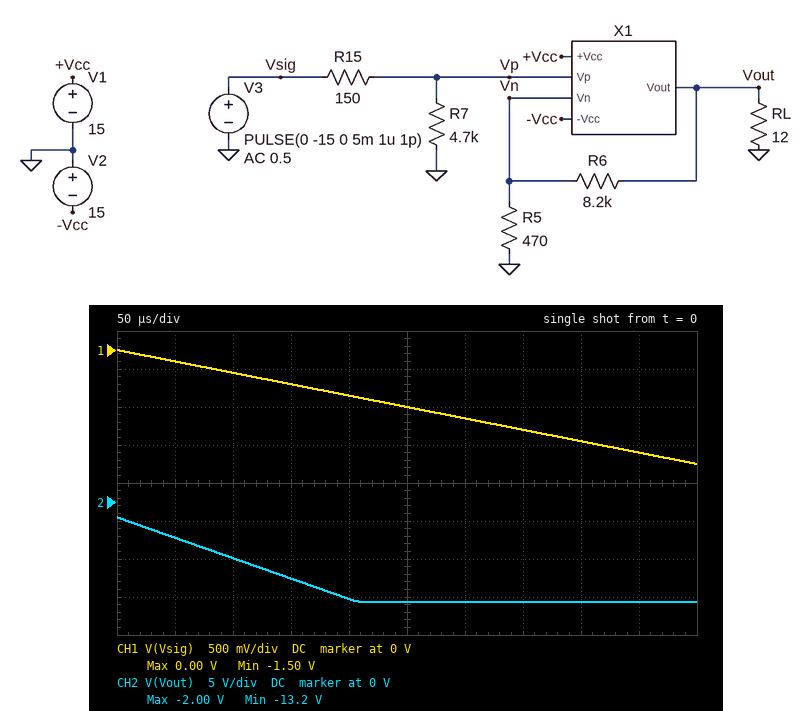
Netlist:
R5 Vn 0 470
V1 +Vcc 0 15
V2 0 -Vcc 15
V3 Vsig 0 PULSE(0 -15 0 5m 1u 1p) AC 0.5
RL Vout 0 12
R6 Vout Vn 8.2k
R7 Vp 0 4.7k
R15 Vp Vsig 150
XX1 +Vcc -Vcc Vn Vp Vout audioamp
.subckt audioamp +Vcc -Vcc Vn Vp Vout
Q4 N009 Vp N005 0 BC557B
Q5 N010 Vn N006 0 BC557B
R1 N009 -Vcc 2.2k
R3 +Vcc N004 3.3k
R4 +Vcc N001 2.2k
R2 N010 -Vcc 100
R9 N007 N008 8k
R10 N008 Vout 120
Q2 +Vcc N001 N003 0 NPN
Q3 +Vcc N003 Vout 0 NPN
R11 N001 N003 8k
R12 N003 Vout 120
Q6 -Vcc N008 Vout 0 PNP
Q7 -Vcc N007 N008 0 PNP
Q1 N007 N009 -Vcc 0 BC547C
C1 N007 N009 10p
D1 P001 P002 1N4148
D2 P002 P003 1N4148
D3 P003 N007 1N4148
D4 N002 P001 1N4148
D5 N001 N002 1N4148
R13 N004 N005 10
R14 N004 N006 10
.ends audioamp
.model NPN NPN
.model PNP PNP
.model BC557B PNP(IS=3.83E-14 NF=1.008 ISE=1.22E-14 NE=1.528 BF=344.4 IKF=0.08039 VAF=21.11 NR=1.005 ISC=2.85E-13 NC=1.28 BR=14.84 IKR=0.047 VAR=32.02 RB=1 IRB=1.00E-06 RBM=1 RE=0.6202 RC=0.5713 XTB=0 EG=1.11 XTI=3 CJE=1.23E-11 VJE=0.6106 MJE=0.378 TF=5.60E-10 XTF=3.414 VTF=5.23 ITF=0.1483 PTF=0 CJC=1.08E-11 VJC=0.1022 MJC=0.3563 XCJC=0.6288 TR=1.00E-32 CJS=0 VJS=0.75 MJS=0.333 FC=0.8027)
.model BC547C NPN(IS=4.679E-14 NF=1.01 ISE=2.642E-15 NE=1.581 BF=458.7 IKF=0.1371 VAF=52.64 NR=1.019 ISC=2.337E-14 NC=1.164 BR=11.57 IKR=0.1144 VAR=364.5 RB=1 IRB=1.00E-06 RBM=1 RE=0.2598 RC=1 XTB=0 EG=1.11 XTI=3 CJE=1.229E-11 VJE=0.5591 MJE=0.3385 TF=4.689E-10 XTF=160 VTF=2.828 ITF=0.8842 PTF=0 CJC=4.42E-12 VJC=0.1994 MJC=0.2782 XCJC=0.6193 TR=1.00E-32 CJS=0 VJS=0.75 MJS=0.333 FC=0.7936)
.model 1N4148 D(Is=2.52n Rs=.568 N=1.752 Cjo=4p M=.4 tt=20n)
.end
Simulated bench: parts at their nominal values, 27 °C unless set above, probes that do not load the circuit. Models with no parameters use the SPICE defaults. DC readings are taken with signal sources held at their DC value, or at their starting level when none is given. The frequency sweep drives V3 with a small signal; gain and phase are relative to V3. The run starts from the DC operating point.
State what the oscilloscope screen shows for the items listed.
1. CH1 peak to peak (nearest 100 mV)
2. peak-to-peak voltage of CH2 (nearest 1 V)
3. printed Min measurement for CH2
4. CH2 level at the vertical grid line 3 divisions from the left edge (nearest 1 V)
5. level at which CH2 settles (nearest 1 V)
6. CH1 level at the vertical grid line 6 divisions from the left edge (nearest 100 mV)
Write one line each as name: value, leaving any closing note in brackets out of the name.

CH1 peak to peak: 1.5 V
peak-to-peak voltage of CH2: 11 V
printed Min measurement for CH2: -13.2 V
CH2 level at the vertical grid line 3 divisions from the left edge: -10 V
level at which CH2 settles: -13 V
CH1 level at the vertical grid line 6 divisions from the left edge: -900 mV
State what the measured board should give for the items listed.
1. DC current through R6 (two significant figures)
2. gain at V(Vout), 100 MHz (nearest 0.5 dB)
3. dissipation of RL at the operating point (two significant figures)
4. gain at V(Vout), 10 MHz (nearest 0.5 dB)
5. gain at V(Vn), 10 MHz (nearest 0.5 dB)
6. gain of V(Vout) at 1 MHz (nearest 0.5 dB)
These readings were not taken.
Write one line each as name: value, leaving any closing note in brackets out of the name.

DC current through R6: 230 µA
gain at V(Vout), 100 MHz: -12.0 dB
dissipation of RL at the operating point: 340 mW
gain at V(Vout), 10 MHz: 22.0 dB
gain at V(Vn), 10 MHz: -7.5 dB
gain of V(Vout) at 1 MHz: 25.0 dB
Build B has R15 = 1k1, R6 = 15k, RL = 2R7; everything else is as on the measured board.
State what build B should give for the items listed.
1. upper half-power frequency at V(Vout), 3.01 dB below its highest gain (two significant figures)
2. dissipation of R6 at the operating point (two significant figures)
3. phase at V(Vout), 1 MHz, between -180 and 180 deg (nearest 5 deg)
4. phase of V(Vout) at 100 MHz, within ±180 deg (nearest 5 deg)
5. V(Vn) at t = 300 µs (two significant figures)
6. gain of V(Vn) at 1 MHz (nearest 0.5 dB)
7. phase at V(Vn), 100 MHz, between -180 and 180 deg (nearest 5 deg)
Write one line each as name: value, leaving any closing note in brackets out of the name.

upper half-power frequency at V(Vout), 3.01 dB below its highest gain: 4.9 MHz
dissipation of R6 at the operating point: 810 µW
phase at V(Vout), 1 MHz, between -180 and 180 deg: -15 deg
phase of V(Vout) at 100 MHz, within ±180 deg: 145 deg
V(Vn) at t = 300 µs: -400 mV
gain of V(Vn) at 1 MHz: -2.0 dB
phase at V(Vn), 100 MHz, between -180 and 180 deg: -5 deg
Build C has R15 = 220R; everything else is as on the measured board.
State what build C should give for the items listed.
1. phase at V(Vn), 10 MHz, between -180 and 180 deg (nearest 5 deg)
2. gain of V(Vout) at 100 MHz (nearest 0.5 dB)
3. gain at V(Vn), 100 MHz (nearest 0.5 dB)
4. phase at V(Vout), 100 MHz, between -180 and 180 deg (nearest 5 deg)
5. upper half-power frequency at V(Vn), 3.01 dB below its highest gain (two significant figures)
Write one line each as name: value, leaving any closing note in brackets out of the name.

phase at V(Vn), 10 MHz, between -180 and 180 deg: -105 deg
gain of V(Vout) at 100 MHz: -13.5 dB
gain at V(Vn), 100 MHz: -7.0 dB
phase at V(Vout), 100 MHz, between -180 and 180 deg: 150 deg
upper half-power frequency at V(Vn), 3.01 dB below its highest gain: 7.1 MHz
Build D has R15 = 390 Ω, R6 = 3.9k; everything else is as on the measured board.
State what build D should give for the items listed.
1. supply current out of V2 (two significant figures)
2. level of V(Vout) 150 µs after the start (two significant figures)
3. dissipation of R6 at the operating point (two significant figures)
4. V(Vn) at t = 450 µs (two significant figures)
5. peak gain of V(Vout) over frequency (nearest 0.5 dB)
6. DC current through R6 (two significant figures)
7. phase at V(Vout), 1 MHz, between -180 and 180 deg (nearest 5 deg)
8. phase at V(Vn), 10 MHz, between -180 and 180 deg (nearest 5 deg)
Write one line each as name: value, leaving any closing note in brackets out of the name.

supply current out of V2: 110 mA
level of V(Vout) 150 µs after the start: -4.9 V
dissipation of R6 at the operating point: 210 µW
V(Vn) at t = 450 µs: -1.4 V
peak gain of V(Vout) over frequency: 21.0 dB
DC current through R6: 230 µA
phase at V(Vout), 1 MHz, between -180 and 180 deg: -5 deg
phase at V(Vn), 10 MHz, between -180 and 180 deg: -80 deg
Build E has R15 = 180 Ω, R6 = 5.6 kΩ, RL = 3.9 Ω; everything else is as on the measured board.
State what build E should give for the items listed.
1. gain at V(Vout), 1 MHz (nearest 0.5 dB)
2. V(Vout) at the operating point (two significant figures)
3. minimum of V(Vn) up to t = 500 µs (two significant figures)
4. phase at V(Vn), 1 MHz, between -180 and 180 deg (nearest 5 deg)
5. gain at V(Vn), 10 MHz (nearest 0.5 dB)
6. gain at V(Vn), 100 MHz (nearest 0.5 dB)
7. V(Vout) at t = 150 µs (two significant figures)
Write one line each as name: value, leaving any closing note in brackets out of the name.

gain at V(Vout), 1 MHz: 22.0 dB
V(Vout) at the operating point: -1.4 V
minimum of V(Vn) up to t = 500 µs: -1.0 V
phase at V(Vn), 1 MHz, between -180 and 180 deg: -5 deg
gain at V(Vn), 10 MHz: -3.5 dB
gain at V(Vn), 100 MHz: -6.0 dB
V(Vout) at t = 150 µs: -7.0 V
